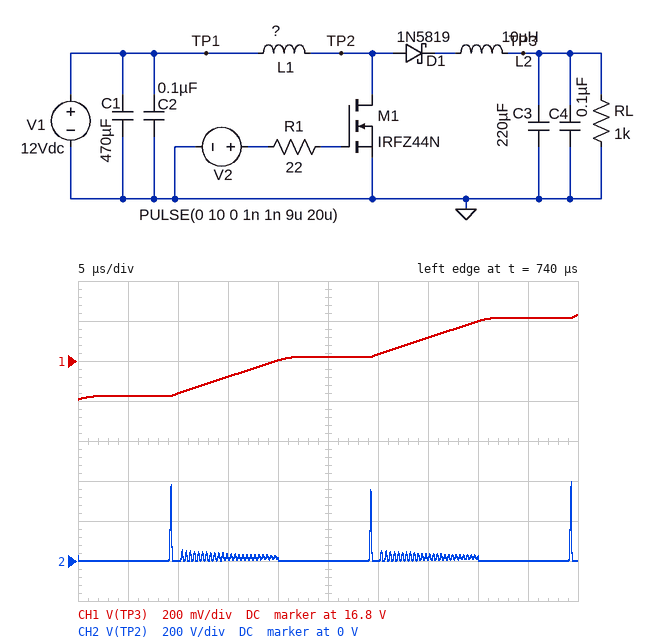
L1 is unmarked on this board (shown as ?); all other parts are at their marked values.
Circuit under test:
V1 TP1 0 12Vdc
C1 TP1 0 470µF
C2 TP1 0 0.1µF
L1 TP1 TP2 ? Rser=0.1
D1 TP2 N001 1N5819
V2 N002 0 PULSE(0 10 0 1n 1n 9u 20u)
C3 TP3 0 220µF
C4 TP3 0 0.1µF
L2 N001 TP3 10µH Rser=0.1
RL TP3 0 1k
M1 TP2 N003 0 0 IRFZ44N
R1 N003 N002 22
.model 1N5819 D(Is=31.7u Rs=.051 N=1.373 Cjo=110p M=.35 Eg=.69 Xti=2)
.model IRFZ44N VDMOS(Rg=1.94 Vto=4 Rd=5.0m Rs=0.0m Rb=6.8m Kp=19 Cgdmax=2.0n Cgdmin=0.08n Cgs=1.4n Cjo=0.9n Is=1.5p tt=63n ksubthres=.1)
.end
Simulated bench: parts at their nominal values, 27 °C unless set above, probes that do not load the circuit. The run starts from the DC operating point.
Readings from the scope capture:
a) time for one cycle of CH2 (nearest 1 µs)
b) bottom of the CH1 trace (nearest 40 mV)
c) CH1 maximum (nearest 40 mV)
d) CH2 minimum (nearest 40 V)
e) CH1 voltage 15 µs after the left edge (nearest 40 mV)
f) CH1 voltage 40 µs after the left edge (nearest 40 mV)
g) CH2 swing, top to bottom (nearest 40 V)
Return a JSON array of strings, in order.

["20 µs", "16.60 V", "17.04 V", "0 V", "16.72 V", "17.00 V", "400 V"]
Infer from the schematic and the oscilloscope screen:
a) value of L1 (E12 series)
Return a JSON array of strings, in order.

["560 µH"]
